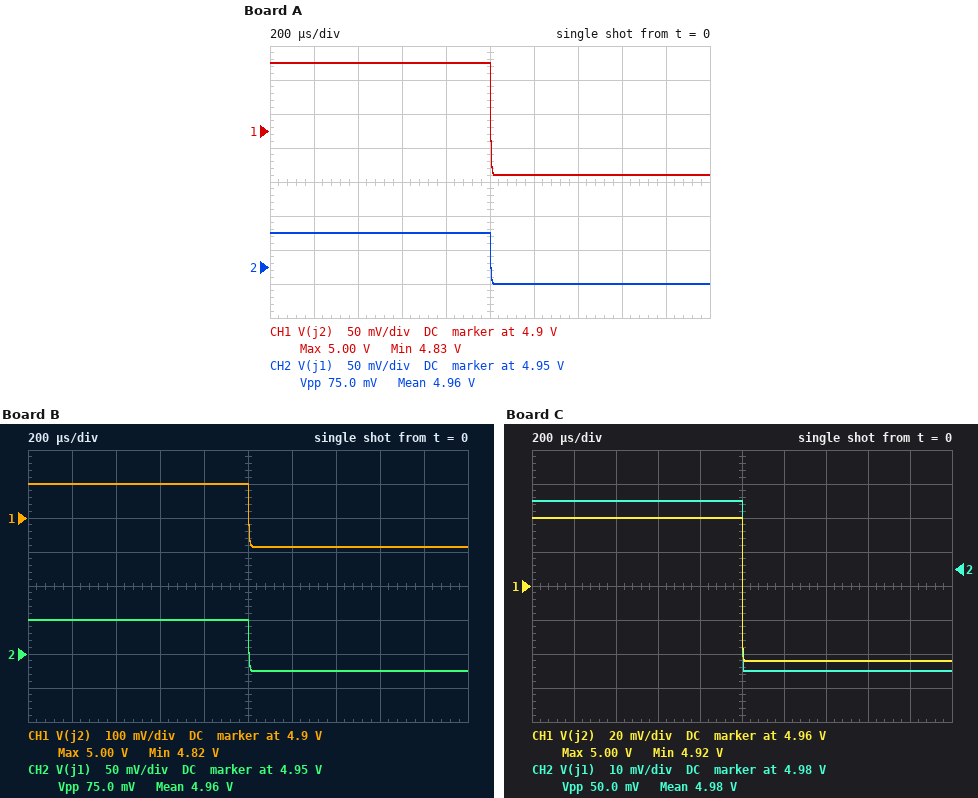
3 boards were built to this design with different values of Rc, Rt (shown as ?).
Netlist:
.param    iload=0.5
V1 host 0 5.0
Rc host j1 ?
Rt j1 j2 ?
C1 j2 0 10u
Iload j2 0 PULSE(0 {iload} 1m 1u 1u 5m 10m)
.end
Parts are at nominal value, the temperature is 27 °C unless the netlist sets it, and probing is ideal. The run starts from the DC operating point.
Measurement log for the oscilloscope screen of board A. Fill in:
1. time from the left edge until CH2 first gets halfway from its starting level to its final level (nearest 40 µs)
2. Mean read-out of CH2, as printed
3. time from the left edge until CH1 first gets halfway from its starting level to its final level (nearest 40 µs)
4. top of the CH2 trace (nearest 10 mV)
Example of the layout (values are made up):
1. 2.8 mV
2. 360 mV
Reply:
1. 1.00 ms
2. 4.96 V
3. 1.00 ms
4. 5.00 V
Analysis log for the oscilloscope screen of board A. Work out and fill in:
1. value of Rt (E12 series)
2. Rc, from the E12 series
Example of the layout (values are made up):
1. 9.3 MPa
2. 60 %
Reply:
1. 0.18 Ω
2. 0.15 Ω
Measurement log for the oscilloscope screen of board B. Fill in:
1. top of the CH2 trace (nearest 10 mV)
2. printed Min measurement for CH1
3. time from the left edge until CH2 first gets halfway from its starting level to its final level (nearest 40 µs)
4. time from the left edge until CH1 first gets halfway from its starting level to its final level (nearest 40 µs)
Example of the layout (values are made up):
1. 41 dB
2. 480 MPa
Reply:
1. 5.00 V
2. 4.82 V
3. 1.00 ms
4. 1.00 ms
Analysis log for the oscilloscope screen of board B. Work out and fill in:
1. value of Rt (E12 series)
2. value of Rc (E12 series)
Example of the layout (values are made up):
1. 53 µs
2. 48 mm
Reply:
1. 0.22 Ω
2. 0.15 Ω
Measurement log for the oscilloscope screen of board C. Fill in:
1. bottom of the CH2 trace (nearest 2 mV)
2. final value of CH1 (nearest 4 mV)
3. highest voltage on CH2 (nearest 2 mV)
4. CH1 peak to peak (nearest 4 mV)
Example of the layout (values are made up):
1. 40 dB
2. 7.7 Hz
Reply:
1. 4.950 V
2. 4.916 V
3. 5.000 V
4. 84 mV
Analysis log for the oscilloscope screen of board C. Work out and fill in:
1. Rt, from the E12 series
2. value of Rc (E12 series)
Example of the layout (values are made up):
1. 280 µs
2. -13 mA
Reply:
1. 0.068 Ω
2. 0.1 Ω
